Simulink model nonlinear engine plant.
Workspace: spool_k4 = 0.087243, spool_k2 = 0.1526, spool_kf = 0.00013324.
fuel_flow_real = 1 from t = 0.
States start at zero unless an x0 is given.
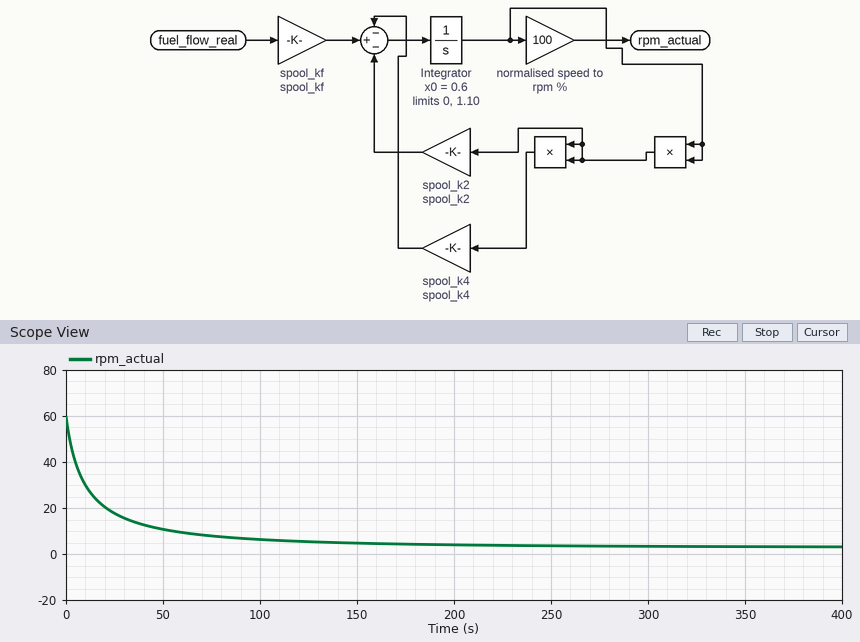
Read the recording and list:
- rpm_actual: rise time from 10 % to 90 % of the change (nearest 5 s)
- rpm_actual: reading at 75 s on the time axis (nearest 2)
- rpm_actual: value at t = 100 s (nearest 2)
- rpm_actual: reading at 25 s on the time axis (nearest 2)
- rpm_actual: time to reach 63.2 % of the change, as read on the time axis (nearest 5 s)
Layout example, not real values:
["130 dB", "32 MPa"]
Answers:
["65 s", "8", "6", "18", "15 s"]
